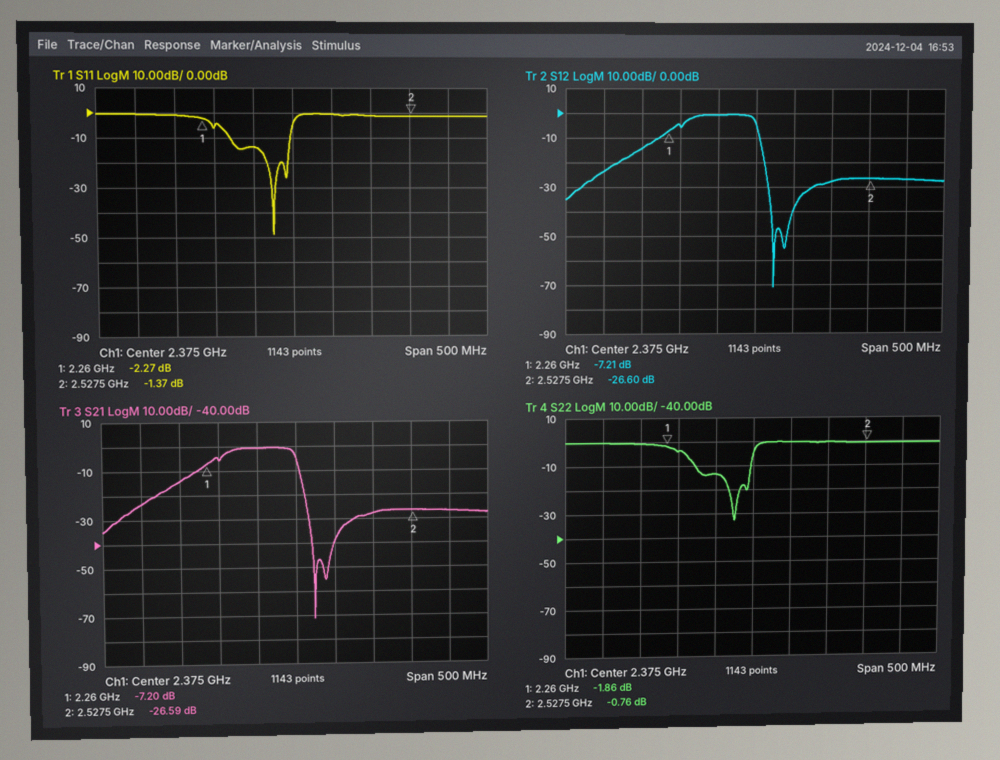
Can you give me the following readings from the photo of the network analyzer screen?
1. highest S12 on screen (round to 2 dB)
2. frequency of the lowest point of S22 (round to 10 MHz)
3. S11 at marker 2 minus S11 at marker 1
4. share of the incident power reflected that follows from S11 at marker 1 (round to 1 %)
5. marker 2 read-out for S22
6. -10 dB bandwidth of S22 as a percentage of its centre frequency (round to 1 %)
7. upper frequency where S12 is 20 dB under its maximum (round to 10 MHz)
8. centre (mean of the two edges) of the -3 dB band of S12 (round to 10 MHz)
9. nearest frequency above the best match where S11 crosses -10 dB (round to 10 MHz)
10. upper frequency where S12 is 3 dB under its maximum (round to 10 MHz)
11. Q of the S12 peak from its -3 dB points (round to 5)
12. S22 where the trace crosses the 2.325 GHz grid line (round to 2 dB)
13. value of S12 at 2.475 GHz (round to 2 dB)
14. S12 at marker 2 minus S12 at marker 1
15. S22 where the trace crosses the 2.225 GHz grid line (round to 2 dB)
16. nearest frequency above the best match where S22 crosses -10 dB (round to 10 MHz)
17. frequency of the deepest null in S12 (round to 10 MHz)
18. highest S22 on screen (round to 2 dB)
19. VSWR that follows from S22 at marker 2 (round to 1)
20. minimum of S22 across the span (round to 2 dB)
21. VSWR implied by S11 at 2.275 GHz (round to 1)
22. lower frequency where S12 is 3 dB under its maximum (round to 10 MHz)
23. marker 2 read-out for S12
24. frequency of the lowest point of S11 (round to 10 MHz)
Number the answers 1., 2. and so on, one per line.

1. 0 dB
2. 2.35 GHz
3. 0.90 dB
4. 59 %
5. -0.76 dB
6. 3 %
7. 2.39 GHz
8. 2.33 GHz
9. 2.37 GHz
10. 2.37 GHz
11. 25
12. -14 dB
13. -28 dB
14. -19.39 dB
15. 0 dB
16. 2.37 GHz
17. 2.40 GHz
18. 0 dB
19. 23
20. -32 dB
21. 3
22. 2.28 GHz
23. -26.60 dB
24. 2.35 GHz
